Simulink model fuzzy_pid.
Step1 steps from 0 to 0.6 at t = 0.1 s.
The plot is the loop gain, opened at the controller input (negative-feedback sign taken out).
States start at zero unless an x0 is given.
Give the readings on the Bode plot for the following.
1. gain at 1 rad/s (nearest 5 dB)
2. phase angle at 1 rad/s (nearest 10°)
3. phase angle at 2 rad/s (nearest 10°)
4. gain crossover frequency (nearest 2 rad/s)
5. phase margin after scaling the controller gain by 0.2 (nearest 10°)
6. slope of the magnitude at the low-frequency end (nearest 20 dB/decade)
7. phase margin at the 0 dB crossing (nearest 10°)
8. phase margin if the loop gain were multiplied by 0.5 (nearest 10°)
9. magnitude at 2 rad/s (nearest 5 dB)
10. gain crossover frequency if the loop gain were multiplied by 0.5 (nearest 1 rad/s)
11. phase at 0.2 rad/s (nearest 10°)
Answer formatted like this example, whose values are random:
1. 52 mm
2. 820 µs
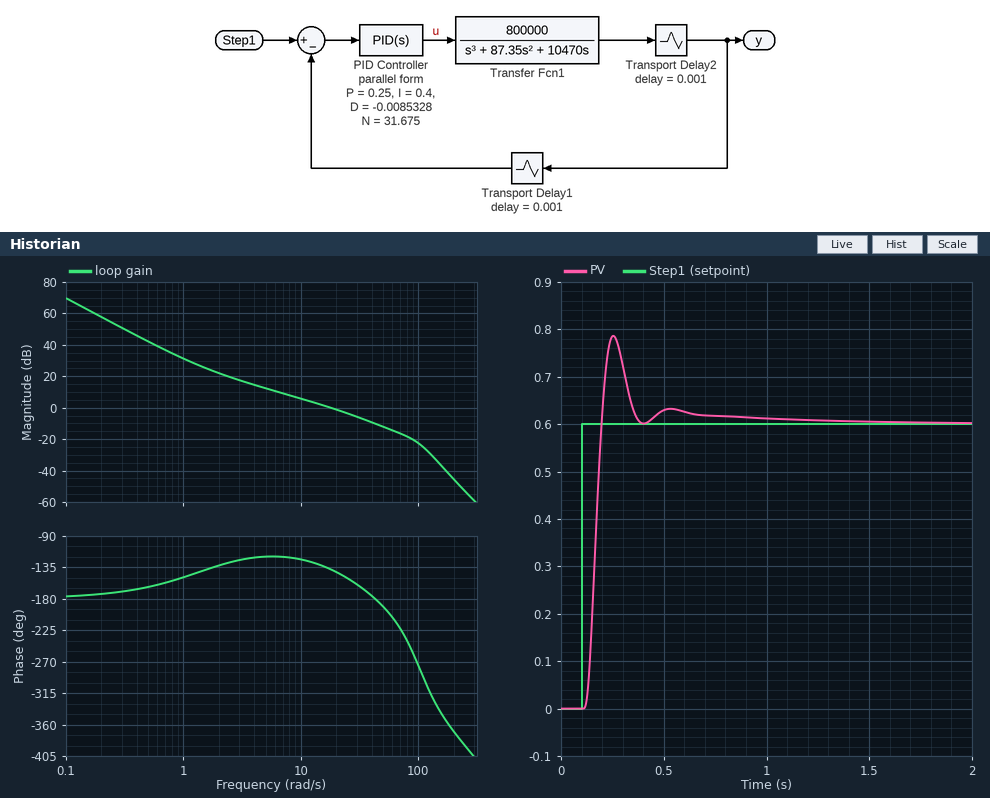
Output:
1. 30 dB
2. -150°
3. -130°
4. 18 rad/s
5. 60°
6. -40 dB/decade
7. 40°
8. 60°
9. 20 dB
10. 10 rad/s
11. -170°
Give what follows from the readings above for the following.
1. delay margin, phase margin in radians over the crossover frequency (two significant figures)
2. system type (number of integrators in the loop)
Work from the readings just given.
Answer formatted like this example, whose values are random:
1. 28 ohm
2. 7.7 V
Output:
1. 0.039 s
2. 2
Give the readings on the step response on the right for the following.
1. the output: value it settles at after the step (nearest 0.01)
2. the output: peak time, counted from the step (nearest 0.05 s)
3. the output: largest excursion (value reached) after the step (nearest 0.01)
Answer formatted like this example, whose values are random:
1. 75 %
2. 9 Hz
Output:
1. 0.60
2. 0.15 s
3. 0.79
